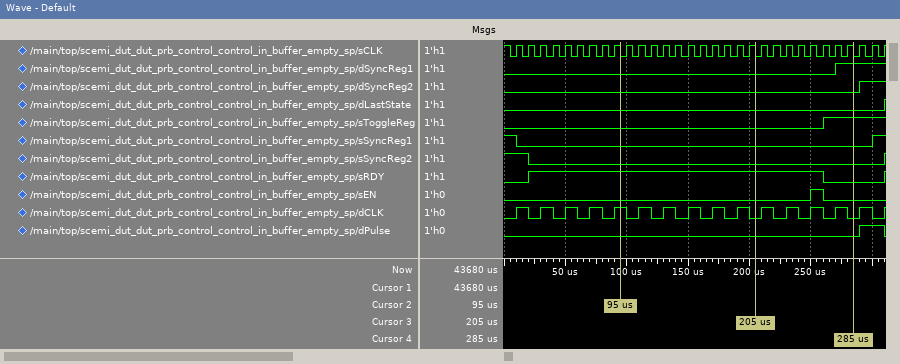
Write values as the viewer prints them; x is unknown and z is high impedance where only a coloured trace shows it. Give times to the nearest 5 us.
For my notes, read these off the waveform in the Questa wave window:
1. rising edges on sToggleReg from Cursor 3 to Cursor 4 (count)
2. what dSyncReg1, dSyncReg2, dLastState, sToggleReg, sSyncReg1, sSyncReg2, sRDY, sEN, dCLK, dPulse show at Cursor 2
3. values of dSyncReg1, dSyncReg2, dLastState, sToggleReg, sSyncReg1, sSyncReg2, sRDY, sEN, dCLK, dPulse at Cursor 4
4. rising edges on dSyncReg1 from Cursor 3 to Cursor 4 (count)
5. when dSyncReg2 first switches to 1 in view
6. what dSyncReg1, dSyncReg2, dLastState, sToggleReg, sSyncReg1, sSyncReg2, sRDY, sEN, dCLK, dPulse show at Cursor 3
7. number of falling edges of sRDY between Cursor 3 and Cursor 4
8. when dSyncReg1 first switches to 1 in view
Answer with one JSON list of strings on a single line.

["1", "dSyncReg1=0, dSyncReg2=0, dLastState=0, sToggleReg=0, sSyncReg1=0, sSyncReg2=0, sRDY=1, sEN=0, dCLK=1, dPulse=0", "dSyncReg1=1, dSyncReg2=0, dLastState=0, sToggleReg=1, sSyncReg1=0, sSyncReg2=0, sRDY=0, sEN=0, dCLK=0, dPulse=0", "1", "290 us", "dSyncReg1=0, dSyncReg2=0, dLastState=0, sToggleReg=0, sSyncReg1=0, sSyncReg2=0, sRDY=1, sEN=0, dCLK=0, dPulse=0", "1", "270 us"]
